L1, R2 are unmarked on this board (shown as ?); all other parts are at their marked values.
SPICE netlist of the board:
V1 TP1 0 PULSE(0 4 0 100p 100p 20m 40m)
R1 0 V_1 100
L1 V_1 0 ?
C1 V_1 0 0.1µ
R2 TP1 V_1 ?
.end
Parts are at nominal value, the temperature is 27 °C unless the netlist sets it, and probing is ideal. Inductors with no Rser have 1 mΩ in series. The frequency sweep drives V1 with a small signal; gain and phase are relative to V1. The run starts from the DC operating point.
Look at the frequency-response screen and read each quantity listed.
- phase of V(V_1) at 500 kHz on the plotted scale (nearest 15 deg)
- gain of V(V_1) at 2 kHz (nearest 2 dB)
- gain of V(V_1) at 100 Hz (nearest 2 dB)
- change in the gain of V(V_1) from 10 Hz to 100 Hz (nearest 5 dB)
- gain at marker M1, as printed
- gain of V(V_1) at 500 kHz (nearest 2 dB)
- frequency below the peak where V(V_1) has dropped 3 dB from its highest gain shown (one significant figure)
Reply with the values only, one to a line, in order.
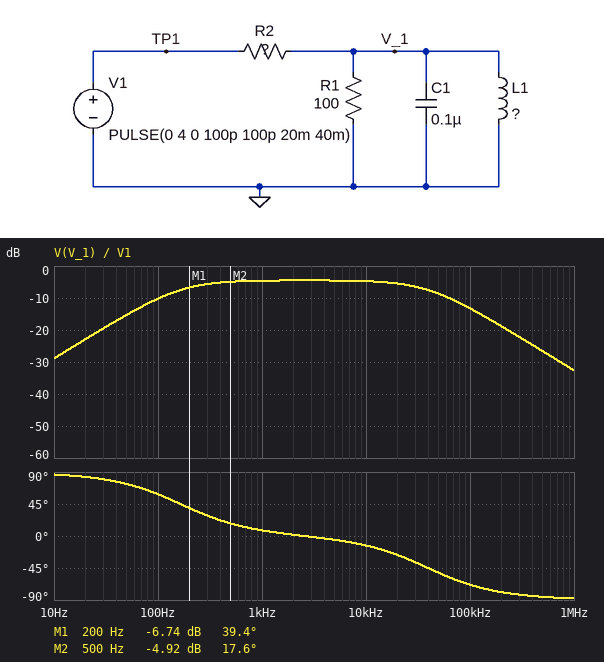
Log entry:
-90 deg
-4 dB
-10 dB
20 dB
-6.74 dB
-26 dB
200 Hz
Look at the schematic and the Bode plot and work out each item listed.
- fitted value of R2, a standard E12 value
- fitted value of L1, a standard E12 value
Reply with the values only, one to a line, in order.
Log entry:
68 Ω
39 mH
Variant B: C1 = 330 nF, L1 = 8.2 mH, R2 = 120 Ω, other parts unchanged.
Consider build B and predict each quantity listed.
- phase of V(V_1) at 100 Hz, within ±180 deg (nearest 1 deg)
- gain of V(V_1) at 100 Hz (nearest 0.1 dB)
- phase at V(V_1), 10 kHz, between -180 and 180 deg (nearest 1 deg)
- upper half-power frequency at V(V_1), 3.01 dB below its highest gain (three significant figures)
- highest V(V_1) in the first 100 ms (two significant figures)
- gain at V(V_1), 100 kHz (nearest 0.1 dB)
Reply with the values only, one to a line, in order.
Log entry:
85 deg
-27.4 dB
-46 deg
9.80 kHz
1.5 V
-27.9 dB
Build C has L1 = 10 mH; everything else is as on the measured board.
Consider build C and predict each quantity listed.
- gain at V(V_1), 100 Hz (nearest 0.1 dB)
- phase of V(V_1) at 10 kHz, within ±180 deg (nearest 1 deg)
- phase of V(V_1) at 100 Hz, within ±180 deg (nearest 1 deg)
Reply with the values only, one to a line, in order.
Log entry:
-20.8 dB
-11 deg
81 deg
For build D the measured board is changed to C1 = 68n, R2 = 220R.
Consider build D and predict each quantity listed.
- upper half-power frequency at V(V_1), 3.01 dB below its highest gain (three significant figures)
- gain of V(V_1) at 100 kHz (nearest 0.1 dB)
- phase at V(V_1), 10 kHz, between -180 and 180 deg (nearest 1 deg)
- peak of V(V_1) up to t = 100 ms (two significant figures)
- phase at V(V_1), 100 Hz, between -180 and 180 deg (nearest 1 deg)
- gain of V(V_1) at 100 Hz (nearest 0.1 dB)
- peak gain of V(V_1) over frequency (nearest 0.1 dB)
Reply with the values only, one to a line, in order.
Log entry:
34.3 kHz
-19.9 dB
-15 deg
1.2 V
70 deg
-19.6 dB
-10.1 dB
